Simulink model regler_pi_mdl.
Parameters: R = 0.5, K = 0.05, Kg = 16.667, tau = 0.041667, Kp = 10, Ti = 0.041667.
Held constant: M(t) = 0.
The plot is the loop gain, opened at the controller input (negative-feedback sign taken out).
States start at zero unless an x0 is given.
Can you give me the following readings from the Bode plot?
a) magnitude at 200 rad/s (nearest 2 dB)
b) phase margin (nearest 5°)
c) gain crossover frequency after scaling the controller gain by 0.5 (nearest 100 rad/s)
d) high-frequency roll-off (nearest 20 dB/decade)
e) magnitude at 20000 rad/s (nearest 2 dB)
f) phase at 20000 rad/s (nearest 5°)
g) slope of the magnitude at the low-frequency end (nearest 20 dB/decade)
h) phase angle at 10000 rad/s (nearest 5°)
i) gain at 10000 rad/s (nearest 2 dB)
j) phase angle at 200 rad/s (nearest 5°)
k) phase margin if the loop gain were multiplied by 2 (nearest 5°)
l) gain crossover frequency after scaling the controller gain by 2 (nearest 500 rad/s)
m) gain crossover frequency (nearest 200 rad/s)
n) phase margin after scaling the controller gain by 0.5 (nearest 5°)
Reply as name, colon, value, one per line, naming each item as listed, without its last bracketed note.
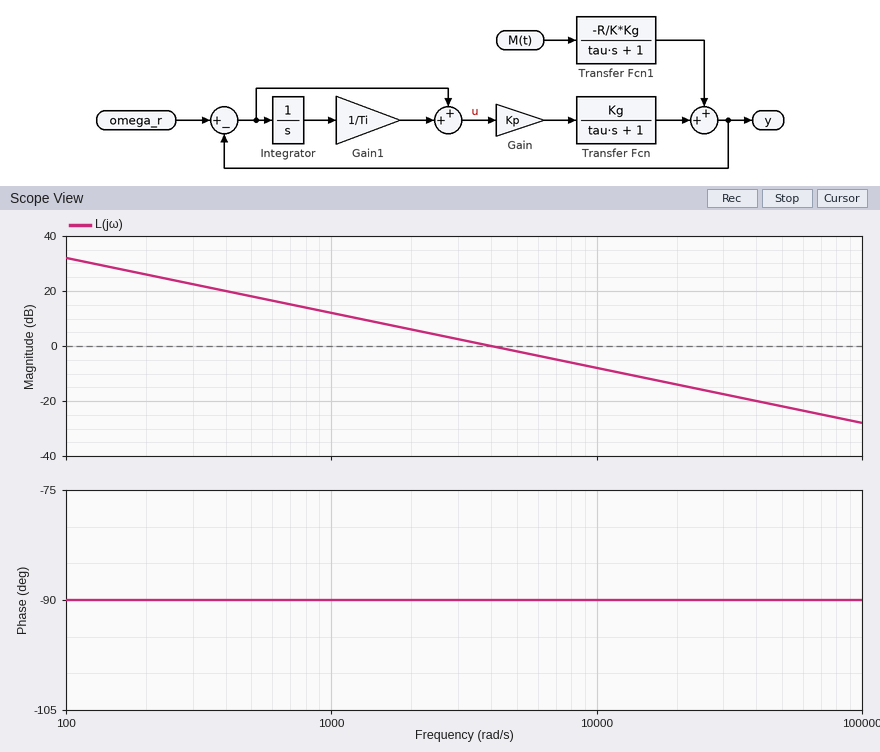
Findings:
magnitude at 200 rad/s: 26 dB
phase margin: 90°
gain crossover frequency after scaling the controller gain by 0.5: 2000 rad/s
high-frequency roll-off: -20 dB/decade
magnitude at 20000 rad/s: -14 dB
phase at 20000 rad/s: -90°
slope of the magnitude at the low-frequency end: -20 dB/decade
phase angle at 10000 rad/s: -90°
gain at 10000 rad/s: -8 dB
phase angle at 200 rad/s: -90°
phase margin if the loop gain were multiplied by 2: 90°
gain crossover frequency after scaling the controller gain by 2: 8000 rad/s
gain crossover frequency: 4000 rad/s
phase margin after scaling the controller gain by 0.5: 90°
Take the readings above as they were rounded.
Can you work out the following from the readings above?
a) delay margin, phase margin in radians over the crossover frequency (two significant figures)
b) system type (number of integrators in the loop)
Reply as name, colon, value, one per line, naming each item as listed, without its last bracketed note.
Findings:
delay margin, phase margin in radians over the crossover frequency: 0.00039 s
system type: 1
